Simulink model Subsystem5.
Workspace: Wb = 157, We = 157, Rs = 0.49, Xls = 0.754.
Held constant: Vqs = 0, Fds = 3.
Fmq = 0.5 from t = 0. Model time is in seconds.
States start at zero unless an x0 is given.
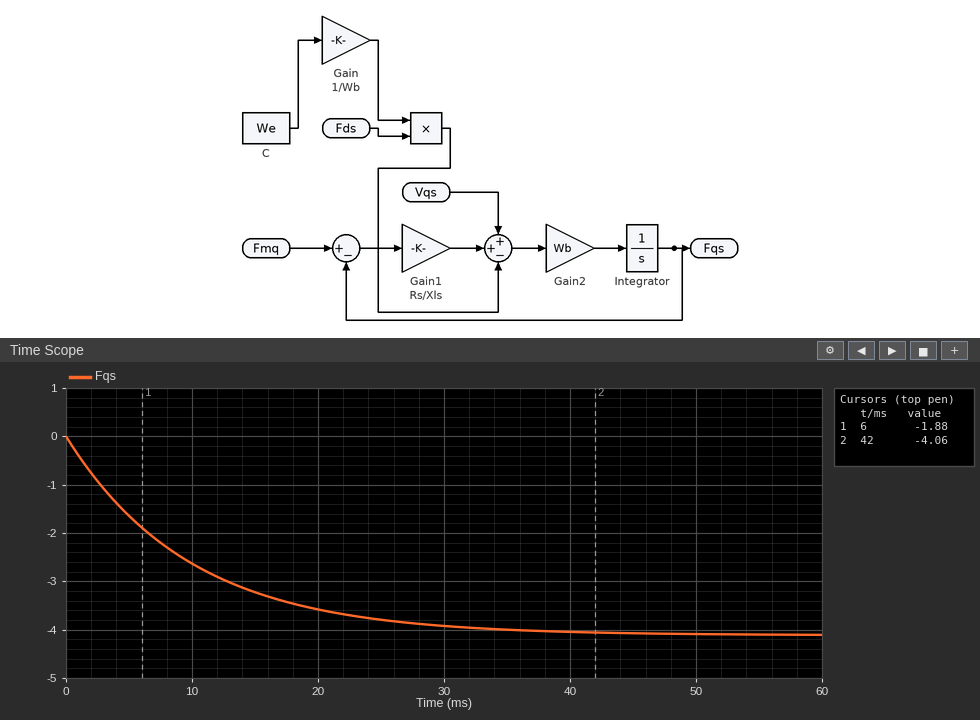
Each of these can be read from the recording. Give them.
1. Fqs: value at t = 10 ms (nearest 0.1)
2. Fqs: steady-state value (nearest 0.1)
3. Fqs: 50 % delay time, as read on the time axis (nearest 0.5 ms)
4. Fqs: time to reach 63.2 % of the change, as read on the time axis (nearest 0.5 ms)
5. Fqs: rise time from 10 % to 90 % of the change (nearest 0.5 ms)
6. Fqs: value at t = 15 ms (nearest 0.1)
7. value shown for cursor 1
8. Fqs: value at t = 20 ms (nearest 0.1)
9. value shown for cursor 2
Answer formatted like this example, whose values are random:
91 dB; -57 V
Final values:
-2.6; -4.1; 7.0 ms; 10.0 ms; 21.5 ms; -3.2; -1.88; -3.6; -4.06
